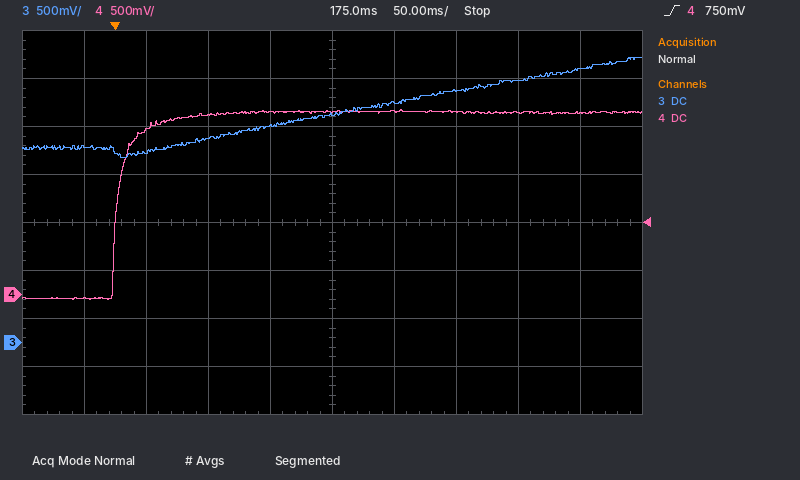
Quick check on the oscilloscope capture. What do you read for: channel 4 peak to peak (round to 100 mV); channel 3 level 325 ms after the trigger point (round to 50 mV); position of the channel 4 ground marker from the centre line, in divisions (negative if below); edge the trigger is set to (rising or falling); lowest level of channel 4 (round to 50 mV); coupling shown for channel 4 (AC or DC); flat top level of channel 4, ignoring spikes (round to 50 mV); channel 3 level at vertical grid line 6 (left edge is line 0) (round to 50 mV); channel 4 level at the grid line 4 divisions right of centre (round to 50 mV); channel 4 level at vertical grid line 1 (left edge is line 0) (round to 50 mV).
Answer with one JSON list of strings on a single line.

["2.00 V", "2.75 V", "-1.5 div", "rising", "-50 mV", "DC", "1.90 V", "2.50 V", "1.90 V", "-50 mV"]
